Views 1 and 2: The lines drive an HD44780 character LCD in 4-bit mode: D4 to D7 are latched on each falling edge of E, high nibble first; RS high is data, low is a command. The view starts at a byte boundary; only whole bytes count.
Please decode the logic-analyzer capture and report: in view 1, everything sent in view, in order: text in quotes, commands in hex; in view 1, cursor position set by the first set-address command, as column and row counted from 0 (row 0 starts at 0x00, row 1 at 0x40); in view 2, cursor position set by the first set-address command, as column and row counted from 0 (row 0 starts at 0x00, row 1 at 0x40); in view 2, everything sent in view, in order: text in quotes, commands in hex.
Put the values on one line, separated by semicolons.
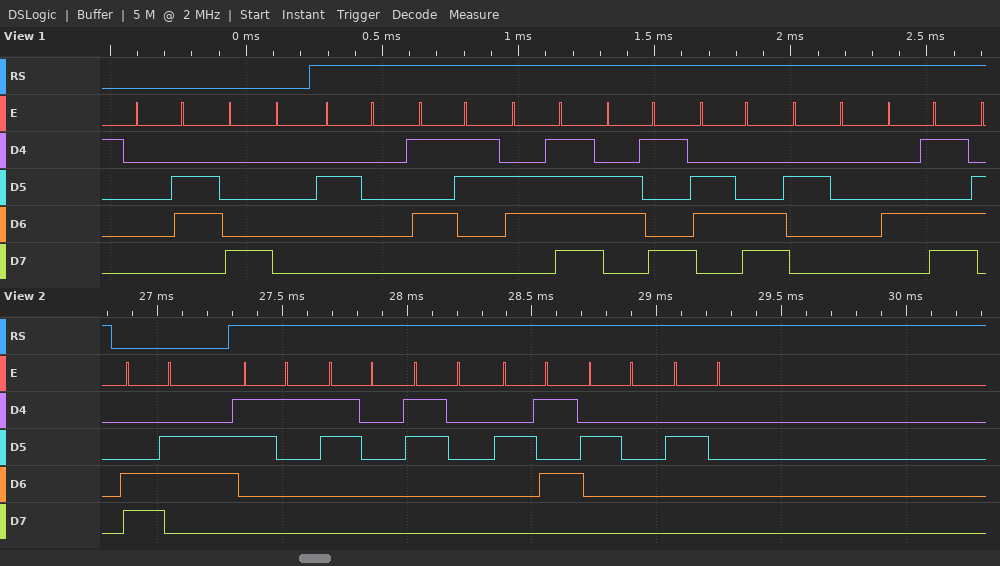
0x06 0x80 " Soil M"; column 0, row 0; column 6, row 1; 0xC6 "100%  "
